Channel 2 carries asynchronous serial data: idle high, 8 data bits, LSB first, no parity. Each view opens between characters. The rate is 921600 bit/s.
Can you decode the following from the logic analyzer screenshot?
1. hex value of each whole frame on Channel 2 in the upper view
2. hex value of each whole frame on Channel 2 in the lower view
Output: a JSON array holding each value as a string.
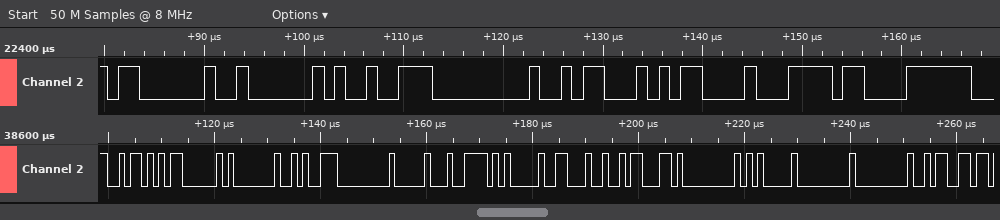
["03, 02, C9, 00, 1A, 0D, BC, F8", "5A, 03, 01, CA, 00, 10, 5E, 90, 24, 63, 00, 05, 00, 00, 9A"]
